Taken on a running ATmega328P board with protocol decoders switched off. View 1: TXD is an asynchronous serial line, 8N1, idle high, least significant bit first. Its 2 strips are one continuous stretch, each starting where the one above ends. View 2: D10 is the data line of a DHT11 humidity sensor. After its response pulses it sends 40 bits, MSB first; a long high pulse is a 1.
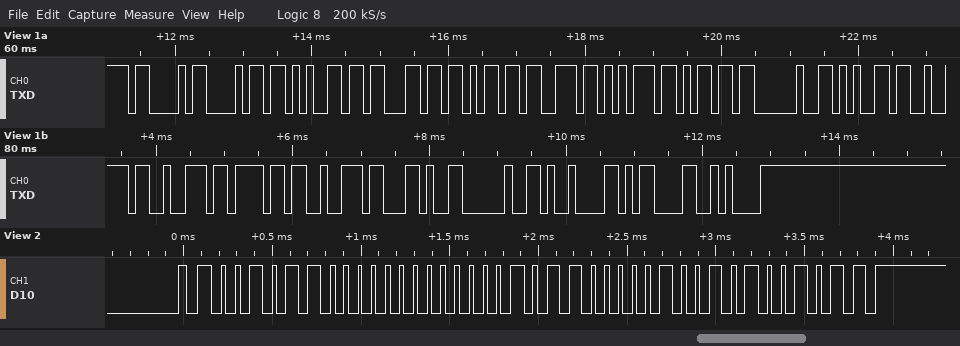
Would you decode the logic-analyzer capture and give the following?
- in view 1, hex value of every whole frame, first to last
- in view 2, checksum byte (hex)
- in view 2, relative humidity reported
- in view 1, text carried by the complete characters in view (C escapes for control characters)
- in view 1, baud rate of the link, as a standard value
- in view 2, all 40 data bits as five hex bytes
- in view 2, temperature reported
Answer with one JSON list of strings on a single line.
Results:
["0x43 0x68 0x65 0x63 0x6B 0x73 0x75 0x6D 0x20 0x65 0x72 0x72 0x6F 0x72 0x2C 0x20 0x09 0x0D 0x0A", "0x4B", "44 %", "\"Checksum error, \\t\\r\\n\"", "9600 baud", "2C 00 16 09 4B", "22.9 °C"]
